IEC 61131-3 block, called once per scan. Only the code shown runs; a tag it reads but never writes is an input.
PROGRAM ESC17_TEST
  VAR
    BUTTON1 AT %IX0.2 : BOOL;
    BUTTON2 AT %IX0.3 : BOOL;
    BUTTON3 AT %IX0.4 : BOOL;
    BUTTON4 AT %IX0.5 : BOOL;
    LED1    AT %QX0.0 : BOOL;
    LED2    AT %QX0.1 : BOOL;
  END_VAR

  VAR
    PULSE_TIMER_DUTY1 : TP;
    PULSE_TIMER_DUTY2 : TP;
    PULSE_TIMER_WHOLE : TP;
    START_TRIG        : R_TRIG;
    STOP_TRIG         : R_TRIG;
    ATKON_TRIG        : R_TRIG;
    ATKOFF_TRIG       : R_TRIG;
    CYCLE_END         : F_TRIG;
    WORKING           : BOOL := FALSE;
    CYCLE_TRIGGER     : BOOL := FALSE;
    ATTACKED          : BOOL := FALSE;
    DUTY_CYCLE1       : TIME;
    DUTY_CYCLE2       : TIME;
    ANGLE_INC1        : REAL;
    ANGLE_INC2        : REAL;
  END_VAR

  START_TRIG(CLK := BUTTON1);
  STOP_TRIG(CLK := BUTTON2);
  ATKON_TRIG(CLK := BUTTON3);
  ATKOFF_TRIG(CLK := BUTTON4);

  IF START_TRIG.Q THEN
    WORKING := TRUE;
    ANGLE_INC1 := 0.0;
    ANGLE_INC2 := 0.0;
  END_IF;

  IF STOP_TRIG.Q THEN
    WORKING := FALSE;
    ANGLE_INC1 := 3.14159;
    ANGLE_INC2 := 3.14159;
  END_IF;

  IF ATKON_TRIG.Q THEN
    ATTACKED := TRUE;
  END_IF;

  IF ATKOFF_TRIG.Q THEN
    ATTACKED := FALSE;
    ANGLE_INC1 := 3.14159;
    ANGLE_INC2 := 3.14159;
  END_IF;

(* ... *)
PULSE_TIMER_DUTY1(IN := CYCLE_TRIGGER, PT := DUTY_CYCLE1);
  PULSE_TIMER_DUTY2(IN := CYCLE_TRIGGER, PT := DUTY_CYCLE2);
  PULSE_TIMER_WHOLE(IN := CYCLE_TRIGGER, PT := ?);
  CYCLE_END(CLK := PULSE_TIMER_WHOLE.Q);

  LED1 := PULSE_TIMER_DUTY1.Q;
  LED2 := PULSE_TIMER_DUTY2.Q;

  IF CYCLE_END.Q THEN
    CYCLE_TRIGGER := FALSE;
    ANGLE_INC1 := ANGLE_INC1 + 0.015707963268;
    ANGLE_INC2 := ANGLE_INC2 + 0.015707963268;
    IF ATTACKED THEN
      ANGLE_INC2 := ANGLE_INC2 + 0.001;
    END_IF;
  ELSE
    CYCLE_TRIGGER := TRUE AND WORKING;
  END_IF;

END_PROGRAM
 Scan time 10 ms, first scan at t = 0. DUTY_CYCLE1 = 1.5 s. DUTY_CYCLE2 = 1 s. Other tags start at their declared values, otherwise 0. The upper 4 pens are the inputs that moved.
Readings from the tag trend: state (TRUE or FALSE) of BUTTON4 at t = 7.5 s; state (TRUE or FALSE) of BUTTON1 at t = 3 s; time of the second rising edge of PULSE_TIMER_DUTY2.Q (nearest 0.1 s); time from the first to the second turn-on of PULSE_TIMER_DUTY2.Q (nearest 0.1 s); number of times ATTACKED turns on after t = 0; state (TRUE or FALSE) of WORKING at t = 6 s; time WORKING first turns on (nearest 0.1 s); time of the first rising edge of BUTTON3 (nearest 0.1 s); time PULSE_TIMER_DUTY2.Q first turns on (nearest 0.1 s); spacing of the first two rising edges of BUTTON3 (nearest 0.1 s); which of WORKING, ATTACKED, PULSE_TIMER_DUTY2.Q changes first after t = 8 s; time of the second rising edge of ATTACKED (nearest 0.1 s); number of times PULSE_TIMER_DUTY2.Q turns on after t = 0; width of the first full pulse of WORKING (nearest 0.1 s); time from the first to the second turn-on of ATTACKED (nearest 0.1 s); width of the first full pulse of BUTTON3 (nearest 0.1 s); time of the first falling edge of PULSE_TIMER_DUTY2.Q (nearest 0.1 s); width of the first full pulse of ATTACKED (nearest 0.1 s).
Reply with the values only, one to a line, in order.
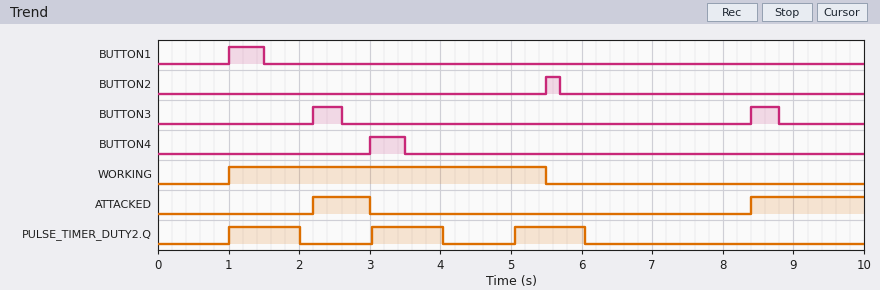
FALSE
FALSE
3.0 s
2.0 s
2
FALSE
1.0 s
2.2 s
1.0 s
6.2 s
ATTACKED
8.4 s
3
4.5 s
6.2 s
0.4 s
2.0 s
0.8 s
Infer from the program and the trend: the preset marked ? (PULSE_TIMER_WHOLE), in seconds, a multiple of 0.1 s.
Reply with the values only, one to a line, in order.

2.0 s
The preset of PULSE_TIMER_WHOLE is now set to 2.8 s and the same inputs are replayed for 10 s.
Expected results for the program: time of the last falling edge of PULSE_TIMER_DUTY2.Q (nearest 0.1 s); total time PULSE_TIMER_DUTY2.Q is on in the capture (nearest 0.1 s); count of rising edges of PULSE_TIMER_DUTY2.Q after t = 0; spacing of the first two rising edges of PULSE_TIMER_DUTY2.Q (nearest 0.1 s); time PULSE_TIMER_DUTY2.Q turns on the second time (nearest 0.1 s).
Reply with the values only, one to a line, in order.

4.8 s
2.0 s
2
2.8 s
3.8 s
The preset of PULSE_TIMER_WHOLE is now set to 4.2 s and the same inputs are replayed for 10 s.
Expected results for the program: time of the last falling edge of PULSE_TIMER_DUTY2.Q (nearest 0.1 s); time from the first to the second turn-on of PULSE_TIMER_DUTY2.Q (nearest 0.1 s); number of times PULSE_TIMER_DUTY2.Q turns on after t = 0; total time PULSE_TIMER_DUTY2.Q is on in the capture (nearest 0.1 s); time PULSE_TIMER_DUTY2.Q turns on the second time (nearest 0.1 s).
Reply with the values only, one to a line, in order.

6.2 s
4.2 s
2
2.0 s
5.2 s
